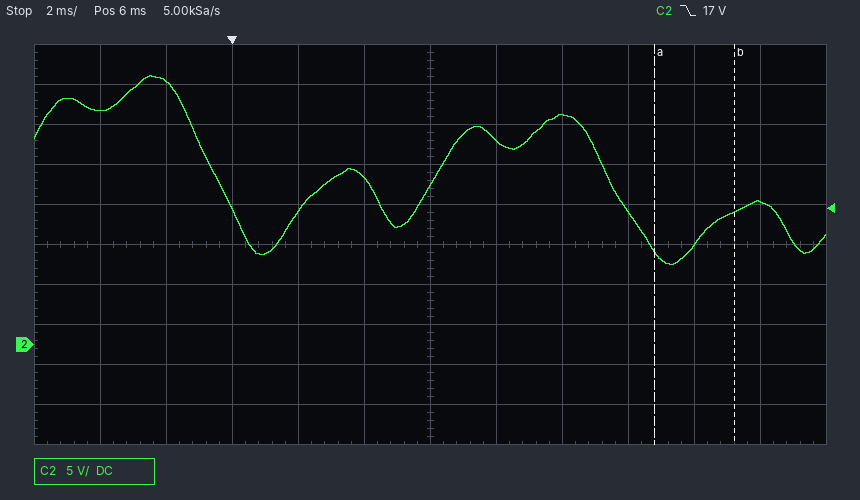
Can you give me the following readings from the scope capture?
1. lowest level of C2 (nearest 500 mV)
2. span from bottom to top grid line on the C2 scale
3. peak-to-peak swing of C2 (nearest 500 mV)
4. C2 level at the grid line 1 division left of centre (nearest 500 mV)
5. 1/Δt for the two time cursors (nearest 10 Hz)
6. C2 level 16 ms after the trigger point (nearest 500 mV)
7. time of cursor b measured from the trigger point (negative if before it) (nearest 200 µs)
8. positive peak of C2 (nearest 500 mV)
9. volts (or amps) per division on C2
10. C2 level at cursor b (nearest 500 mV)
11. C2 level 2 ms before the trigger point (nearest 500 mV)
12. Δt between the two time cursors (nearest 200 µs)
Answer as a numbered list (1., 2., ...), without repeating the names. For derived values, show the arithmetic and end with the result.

1. 10.0 V
2. 50 V
3. 33.5 V − (10.0 V) = 23.5 V
4. 21.0 V
5. 1 / 2.4 ms ≈ 420 Hz
6. 18.0 V
7. +15.2 ms
8. 33.5 V
9. 5 V
10. 16.5 V
11. 33.0 V
12. 2.4 ms
